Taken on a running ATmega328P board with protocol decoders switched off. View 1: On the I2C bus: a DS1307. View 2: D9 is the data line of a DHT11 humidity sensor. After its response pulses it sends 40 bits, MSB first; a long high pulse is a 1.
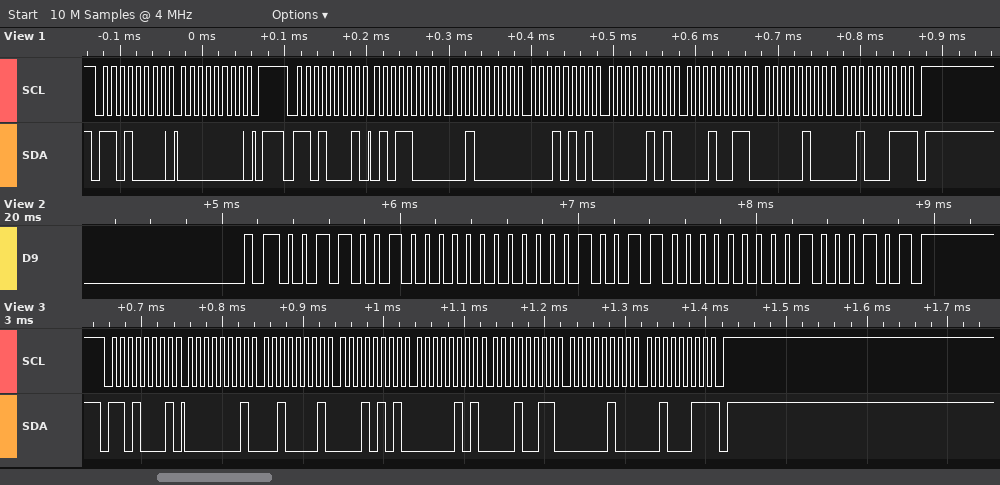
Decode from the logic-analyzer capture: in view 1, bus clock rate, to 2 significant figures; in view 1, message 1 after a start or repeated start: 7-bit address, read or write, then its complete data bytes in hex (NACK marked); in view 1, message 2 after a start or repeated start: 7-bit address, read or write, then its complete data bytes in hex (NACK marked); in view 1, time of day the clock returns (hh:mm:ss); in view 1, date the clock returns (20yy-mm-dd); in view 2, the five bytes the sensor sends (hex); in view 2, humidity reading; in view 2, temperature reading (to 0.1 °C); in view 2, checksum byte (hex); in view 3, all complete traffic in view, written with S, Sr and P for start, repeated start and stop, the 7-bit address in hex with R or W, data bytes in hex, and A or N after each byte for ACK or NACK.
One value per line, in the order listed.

100 kHz
0x68 write: 00
0x68 read: 58 20 15 05 13 04 23 NACK
15:20:58
2023-04-13
32 00 13 00 45
50 %
19.0 °C
0x45
S 68R A 01 A 21 A 15 A 05 A 13 A 04 A 23 N P
